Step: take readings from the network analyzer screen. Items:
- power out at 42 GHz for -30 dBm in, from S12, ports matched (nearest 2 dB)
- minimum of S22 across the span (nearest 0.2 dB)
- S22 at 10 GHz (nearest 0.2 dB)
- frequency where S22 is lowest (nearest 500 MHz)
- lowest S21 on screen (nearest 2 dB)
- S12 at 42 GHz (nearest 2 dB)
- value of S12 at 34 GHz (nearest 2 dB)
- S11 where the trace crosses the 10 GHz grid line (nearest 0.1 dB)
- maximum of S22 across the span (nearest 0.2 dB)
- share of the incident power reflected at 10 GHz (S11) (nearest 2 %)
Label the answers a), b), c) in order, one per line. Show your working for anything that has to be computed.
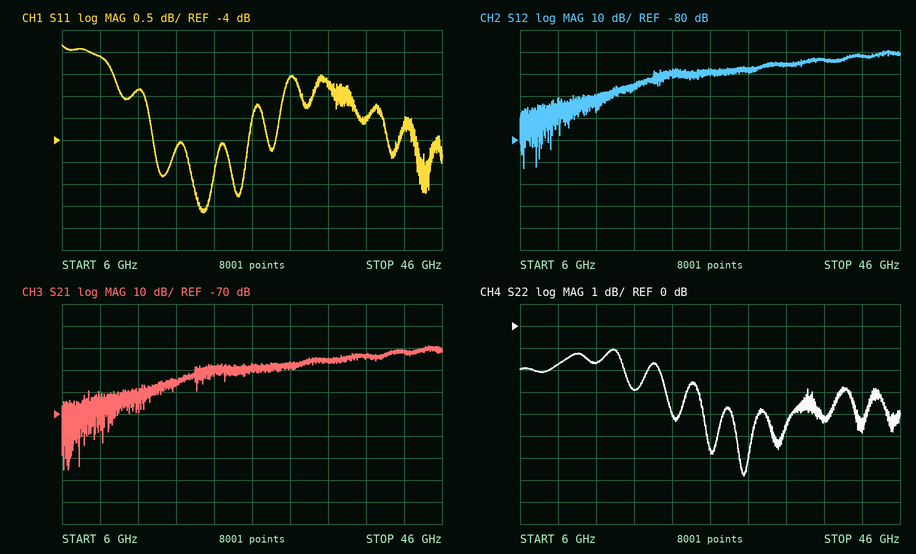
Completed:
a) -30 dBm + (-42 dB) = -72 dBm
b) -6.8 dB
c) -1.8 dB
d) 29.5 GHz
e) -96 dB
f) -42 dB
g) -46 dB
h) -2.1 dB
i) -1.0 dB
j) 10^(-2.1/10) ≈ 62 %
